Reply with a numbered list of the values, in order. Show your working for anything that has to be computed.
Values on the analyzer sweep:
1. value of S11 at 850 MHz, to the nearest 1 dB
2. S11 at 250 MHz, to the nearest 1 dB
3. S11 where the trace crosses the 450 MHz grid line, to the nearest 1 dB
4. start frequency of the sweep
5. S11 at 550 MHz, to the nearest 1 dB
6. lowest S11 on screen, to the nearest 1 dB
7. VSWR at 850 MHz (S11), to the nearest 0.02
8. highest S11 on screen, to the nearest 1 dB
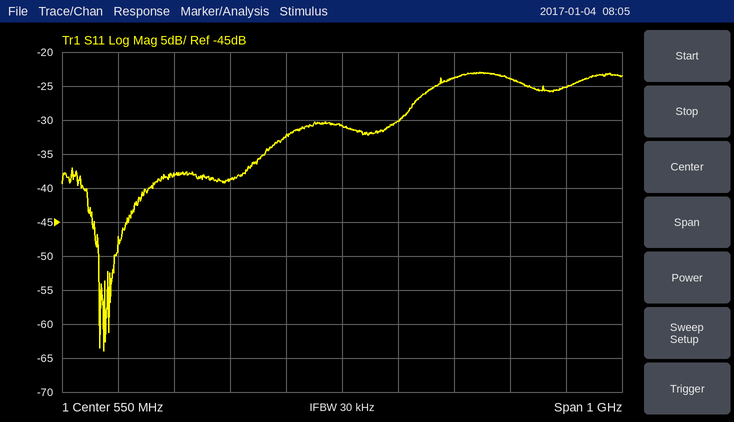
1. -24 dB
2. -38 dB
3. -32 dB
4. 50 MHz
5. -31 dB
6. -64 dB
7. |Γ| = 10^(-24/20) = 0.0631; VSWR = (1 + 0.0631)/(1 − 0.0631) ≈ 1.13, so 1.14 to the nearest 0.02
8. -23 dB
